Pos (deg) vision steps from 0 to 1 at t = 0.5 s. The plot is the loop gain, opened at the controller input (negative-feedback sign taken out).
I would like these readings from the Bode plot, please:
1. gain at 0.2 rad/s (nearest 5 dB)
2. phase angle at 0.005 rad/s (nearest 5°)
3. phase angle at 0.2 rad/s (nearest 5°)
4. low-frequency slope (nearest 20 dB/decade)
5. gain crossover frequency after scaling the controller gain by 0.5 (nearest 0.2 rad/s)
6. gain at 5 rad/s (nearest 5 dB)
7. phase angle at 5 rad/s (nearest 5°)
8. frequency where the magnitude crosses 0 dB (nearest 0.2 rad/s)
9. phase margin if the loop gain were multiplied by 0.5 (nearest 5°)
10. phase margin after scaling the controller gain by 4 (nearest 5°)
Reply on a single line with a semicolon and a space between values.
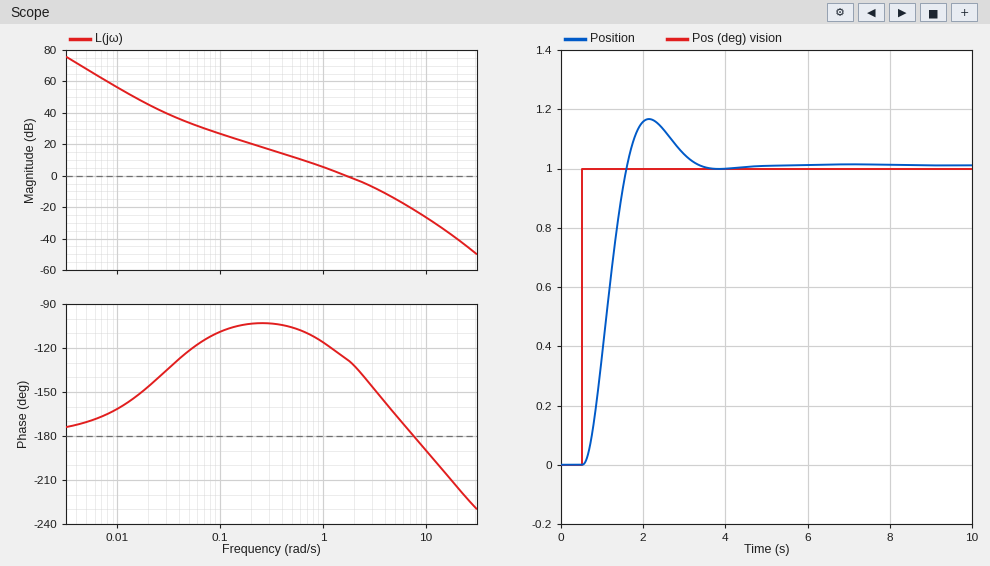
20 dB; -170°; -105°; -40 dB/decade; 1.0 rad/s; -15 dB; -165°; 1.6 rad/s; 65°; 20°
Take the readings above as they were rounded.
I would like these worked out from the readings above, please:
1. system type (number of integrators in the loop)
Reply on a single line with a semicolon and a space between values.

2
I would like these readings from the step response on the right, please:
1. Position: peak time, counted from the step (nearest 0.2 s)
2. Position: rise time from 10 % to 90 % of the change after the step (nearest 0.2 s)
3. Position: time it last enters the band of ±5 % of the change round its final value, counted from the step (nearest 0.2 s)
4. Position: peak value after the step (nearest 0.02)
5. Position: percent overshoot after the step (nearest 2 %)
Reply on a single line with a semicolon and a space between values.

1.6 s; 0.8 s; 2.4 s; 1.16; 16 %
